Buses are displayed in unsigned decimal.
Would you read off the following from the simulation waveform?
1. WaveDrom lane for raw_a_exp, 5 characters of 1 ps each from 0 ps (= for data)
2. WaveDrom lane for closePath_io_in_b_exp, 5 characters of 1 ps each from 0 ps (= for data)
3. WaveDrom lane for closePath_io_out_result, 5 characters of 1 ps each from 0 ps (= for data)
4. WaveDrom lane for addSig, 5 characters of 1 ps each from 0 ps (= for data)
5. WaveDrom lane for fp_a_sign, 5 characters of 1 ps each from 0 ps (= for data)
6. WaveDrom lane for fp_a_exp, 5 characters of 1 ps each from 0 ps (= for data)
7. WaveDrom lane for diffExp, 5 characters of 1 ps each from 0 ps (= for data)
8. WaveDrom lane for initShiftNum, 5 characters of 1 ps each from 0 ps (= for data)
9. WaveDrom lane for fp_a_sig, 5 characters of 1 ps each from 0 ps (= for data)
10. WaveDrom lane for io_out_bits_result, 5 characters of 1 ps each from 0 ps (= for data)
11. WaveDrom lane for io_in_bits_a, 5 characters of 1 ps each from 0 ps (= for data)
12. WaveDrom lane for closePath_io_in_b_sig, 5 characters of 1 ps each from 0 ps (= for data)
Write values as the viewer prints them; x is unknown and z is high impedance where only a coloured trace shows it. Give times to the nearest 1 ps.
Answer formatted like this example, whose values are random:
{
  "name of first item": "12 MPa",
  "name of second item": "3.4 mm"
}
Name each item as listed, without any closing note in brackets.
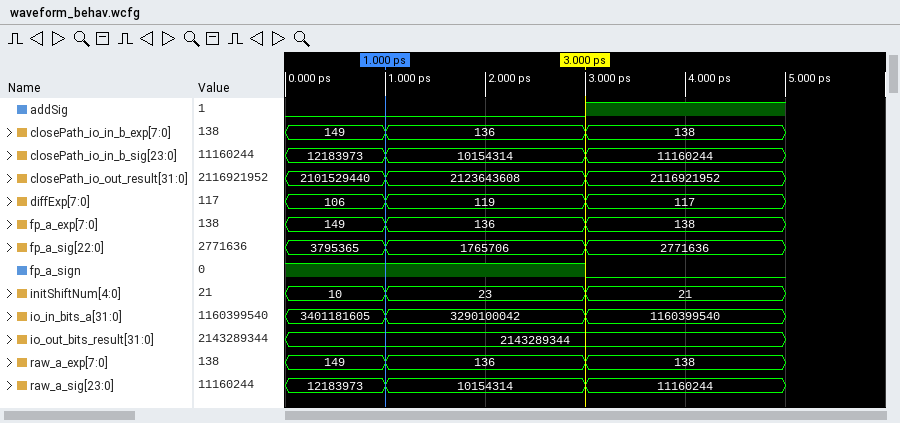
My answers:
{
  "WaveDrom lane for raw_a_exp, 5 characters of 1 ps each from 0 ps": "{name: 'raw_a_exp', wave: '==.=.', data: '149 136 138'}",
  "WaveDrom lane for closePath_io_in_b_exp, 5 characters of 1 ps each from 0 ps": "{name: 'closePath_io_in_b_exp', wave: '==.=.', data: '149 136 138'}",
  "WaveDrom lane for closePath_io_out_result, 5 characters of 1 ps each from 0 ps": "{name: 'closePath_io_out_result', wave: '==.=.', data: '2101529440 2123643608 2116921952'}",
  "WaveDrom lane for addSig, 5 characters of 1 ps each from 0 ps": "{name: 'addSig', wave: '0..1.'}",
  "WaveDrom lane for fp_a_sign, 5 characters of 1 ps each from 0 ps": "{name: 'fp_a_sign', wave: '1..0.'}",
  "WaveDrom lane for fp_a_exp, 5 characters of 1 ps each from 0 ps": "{name: 'fp_a_exp', wave: '==.=.', data: '149 136 138'}",
  "WaveDrom lane for diffExp, 5 characters of 1 ps each from 0 ps": "{name: 'diffExp', wave: '==.=.', data: '106 119 117'}",
  "WaveDrom lane for initShiftNum, 5 characters of 1 ps each from 0 ps": "{name: 'initShiftNum', wave: '==.=.', data: '10 23 21'}",
  "WaveDrom lane for fp_a_sig, 5 characters of 1 ps each from 0 ps": "{name: 'fp_a_sig', wave: '==.=.', data: '3795365 1765706 2771636'}",
  "WaveDrom lane for io_out_bits_result, 5 characters of 1 ps each from 0 ps": "{name: 'io_out_bits_result', wave: '=....', data: '2143289344'}",
  "WaveDrom lane for io_in_bits_a, 5 characters of 1 ps each from 0 ps": "{name: 'io_in_bits_a', wave: '==.=.', data: '3401181605 3290100042 1160399540'}",
  "WaveDrom lane for closePath_io_in_b_sig, 5 characters of 1 ps each from 0 ps": "{name: 'closePath_io_in_b_sig', wave: '==.=.', data: '12183973 10154314 11160244'}"
}
